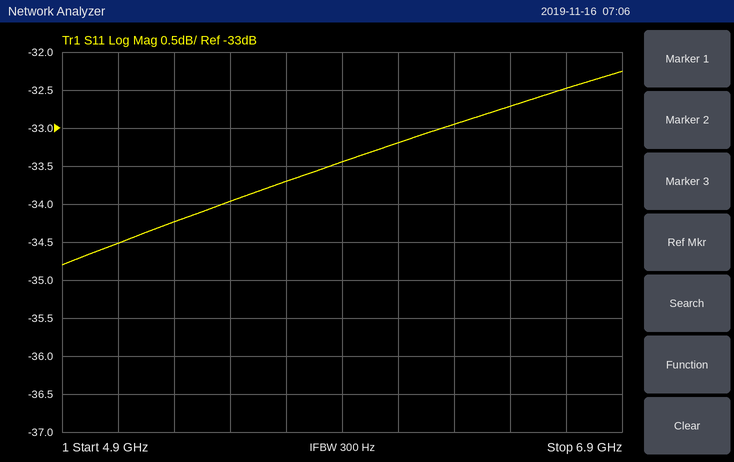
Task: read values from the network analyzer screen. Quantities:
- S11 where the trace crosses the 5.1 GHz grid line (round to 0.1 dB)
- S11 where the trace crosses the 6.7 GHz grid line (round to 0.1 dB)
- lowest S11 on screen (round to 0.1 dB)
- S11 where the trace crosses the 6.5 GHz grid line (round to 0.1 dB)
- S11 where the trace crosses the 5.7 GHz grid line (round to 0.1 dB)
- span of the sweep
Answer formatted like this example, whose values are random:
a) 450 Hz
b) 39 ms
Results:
a) -34.5 dB
b) -32.5 dB
c) -34.8 dB
d) -32.7 dB
e) -33.7 dB
f) 2 GHz
